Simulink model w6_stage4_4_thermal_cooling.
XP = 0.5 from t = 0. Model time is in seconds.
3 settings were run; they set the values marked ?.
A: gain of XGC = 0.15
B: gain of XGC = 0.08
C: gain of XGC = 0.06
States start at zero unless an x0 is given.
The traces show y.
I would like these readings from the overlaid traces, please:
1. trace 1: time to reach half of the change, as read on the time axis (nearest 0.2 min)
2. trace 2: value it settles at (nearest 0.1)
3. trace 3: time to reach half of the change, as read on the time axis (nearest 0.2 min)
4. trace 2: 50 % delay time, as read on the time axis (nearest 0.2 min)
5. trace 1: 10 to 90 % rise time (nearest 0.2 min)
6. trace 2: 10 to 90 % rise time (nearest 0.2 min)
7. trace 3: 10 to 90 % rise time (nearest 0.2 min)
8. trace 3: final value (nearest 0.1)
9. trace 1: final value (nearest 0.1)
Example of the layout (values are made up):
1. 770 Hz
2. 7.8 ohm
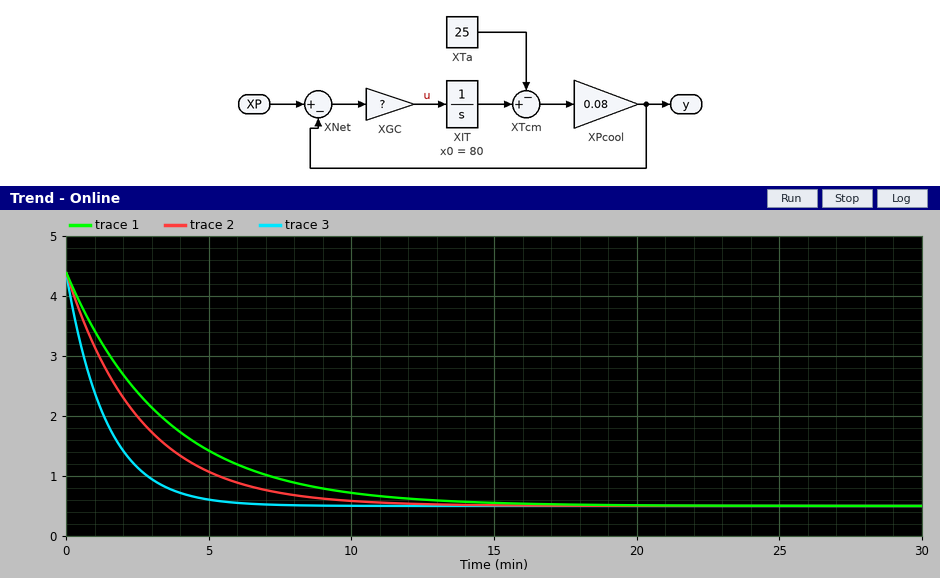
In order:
1. 2.4 min
2. 0.5
3. 1.0 min
4. 1.8 min
5. 7.6 min
6. 5.8 min
7. 3.0 min
8. 0.5
9. 0.5
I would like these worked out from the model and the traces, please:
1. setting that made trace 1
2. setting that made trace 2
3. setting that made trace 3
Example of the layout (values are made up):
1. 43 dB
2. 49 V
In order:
1. C
2. B
3. A
